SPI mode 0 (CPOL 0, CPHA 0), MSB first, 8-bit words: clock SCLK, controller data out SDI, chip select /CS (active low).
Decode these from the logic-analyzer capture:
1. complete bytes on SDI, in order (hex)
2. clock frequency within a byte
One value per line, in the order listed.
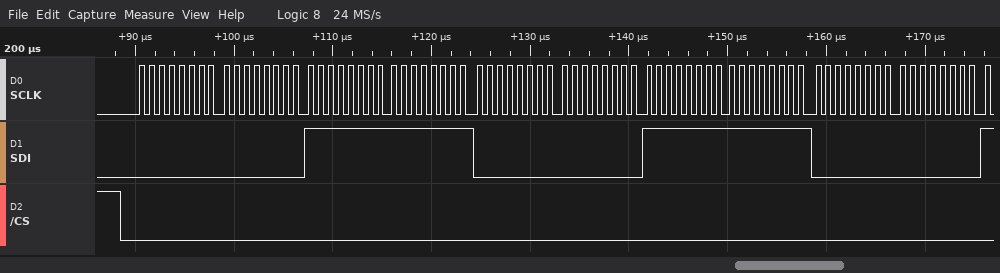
0x00 0x00 0xFF 0xFF 0x00 0x00 0xFF 0xFF 0x00 0x00
1 MHz
